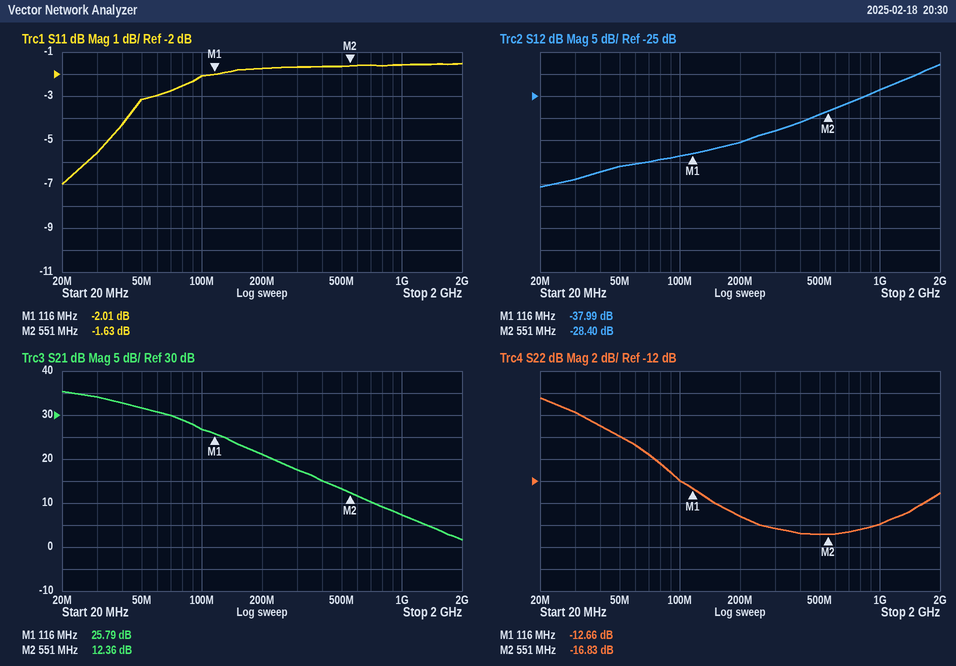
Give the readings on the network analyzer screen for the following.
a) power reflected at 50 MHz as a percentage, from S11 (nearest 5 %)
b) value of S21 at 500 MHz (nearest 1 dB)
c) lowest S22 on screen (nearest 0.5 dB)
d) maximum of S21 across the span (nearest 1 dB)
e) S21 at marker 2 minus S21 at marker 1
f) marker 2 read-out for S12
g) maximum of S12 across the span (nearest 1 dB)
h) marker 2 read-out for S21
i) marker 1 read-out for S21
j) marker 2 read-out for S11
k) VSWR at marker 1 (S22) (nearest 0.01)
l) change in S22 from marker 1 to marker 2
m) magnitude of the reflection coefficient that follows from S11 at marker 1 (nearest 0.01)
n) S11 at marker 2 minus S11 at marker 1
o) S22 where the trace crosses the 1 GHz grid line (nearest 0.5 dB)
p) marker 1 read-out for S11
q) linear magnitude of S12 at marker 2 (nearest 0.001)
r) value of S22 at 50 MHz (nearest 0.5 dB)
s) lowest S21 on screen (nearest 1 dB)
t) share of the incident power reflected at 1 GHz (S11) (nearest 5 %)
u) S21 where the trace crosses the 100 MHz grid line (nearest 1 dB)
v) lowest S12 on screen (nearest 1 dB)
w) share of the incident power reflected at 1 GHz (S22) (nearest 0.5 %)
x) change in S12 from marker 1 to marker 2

50 %
13 dB
-17.0 dB
35 dB
-13.43 dB
-28.40 dB
-18 dB
12.36 dB
25.79 dB
-1.63 dB
1.61
-4.17 dB
0.79
0.38 dB
-16.0 dB
-2.01 dB
0.038
-8.0 dB
2 dB
70 %
27 dB
-46 dB
2.5 %
9.59 dB
